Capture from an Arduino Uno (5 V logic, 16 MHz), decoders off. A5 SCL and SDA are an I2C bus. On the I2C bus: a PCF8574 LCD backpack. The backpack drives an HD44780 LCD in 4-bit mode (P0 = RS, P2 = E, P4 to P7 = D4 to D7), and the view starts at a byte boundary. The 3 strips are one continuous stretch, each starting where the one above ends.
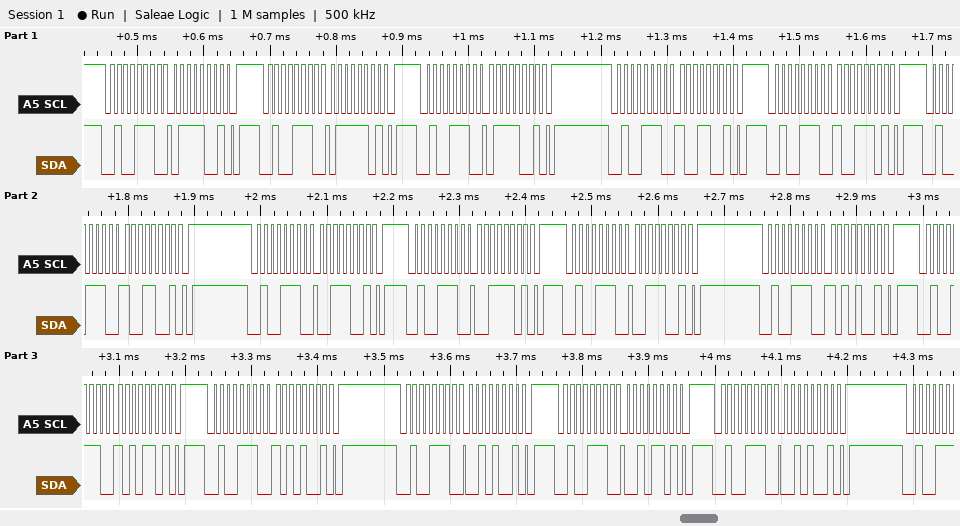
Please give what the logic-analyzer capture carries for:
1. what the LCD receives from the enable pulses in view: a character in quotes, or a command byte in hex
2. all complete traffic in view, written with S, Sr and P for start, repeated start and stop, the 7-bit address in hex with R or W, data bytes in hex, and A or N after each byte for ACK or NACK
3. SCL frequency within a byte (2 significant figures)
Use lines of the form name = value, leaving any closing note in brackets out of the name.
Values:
what the LCD receives from the enable pulses in view: a character in quotes, or a command byte in hex = 'y' ':'
all complete traffic in view, written with S, Sr and P for start, repeated start and stop, the 7-bit address in hex with R or W, data bytes in hex, and A or N after each byte for ACK or NACK = S 27W A 79 A P S 27W A 7D A P S 27W A 79 A P S 27W A 99 A P S 27W A 9D A P S 27W A 99 A P S 27W A 39 A P S 27W A 3D A P S 27W A 39 A P S 27W A A9 A P S 27W A AD A P S 27W A A9 A P S 27W A 29 A P S 27W A 2D A P S 27W A 29 A P
SCL frequency within a byte = 100 kHz
